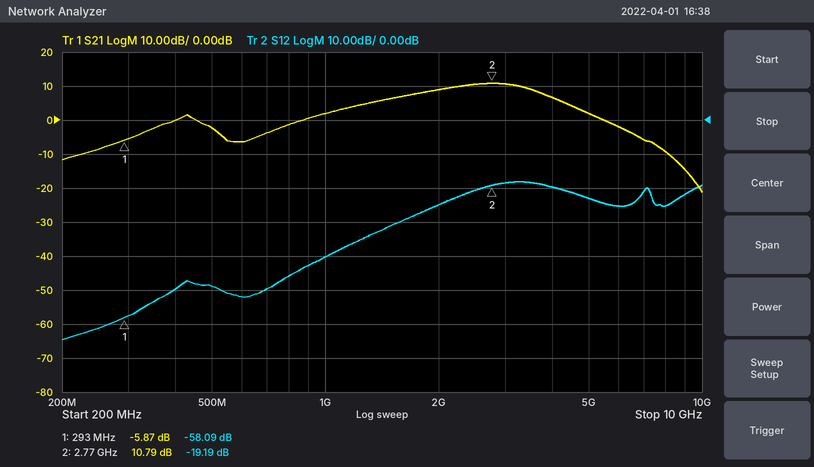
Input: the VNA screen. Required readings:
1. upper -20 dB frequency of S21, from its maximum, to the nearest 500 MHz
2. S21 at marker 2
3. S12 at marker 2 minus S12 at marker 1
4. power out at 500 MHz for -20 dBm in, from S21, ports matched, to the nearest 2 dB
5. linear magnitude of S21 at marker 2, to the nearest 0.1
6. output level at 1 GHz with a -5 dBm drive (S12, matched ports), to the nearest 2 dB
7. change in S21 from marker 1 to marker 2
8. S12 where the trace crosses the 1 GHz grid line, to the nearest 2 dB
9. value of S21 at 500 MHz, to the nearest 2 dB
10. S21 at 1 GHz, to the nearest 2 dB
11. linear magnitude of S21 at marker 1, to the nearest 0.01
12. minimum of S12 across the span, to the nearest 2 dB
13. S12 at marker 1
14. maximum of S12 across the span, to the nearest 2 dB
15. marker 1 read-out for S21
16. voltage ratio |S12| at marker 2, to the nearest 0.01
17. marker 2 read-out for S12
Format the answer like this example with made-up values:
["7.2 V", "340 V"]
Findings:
["8.0 GHz", "10.79 dB", "38.90 dB", "-22 dBm", "3.5", "-46 dBm", "16.66 dB", "-40 dB", "-2 dB", "2 dB", "0.51", "-64 dB", "-58.09 dB", "-18 dB", "-5.87 dB", "0.11", "-19.19 dB"]
